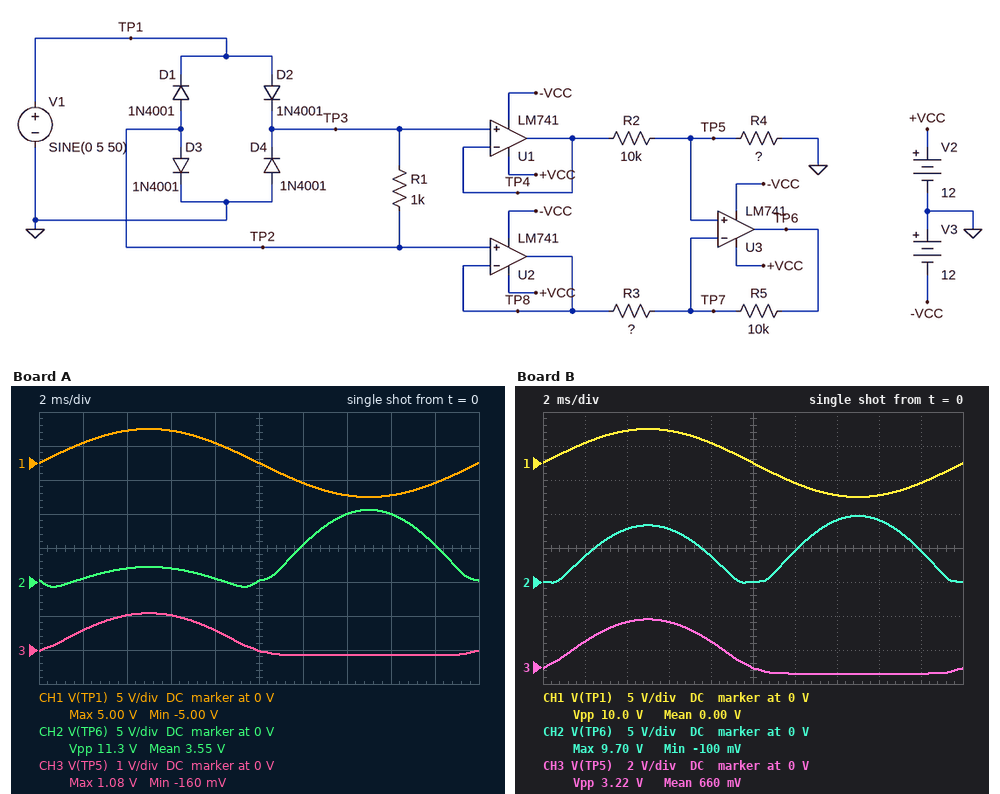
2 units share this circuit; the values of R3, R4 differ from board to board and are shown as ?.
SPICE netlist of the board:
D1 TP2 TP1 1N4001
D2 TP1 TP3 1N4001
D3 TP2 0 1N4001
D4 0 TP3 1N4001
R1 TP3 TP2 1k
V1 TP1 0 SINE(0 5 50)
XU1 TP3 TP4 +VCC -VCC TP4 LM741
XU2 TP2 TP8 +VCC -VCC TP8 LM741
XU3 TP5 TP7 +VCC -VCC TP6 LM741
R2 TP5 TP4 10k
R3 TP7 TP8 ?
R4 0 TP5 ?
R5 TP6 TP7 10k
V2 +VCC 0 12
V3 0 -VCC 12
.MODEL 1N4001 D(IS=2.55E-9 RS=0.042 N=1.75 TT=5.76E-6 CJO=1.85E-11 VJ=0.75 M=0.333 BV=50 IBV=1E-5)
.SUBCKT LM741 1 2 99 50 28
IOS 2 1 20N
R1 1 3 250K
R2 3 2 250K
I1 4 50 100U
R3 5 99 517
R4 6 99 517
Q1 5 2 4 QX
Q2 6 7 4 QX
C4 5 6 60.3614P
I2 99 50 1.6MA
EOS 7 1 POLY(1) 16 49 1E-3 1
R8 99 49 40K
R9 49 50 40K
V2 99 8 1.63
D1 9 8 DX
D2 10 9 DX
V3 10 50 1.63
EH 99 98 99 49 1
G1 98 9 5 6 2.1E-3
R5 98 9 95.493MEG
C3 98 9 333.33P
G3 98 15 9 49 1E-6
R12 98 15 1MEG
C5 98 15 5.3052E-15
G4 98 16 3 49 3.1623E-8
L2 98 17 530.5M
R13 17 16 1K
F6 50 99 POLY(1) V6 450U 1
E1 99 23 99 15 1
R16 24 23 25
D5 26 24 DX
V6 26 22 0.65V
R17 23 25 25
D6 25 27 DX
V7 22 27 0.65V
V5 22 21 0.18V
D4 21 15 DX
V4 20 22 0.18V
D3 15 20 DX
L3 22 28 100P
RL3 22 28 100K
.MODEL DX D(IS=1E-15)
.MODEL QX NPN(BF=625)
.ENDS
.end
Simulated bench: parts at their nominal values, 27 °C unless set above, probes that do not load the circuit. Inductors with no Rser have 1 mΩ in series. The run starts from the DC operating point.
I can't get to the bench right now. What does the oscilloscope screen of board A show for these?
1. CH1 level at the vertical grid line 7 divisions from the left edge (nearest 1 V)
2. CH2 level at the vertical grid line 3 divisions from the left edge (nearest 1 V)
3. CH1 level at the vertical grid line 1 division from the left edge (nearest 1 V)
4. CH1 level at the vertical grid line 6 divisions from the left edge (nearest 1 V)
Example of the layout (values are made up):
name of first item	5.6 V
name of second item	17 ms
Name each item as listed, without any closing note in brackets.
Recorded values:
CH1 level at the vertical grid line 7 divisions from the left edge	-5 V
CH2 level at the vertical grid line 3 divisions from the left edge	2 V
CH1 level at the vertical grid line 1 division from the left edge	3 V
CH1 level at the vertical grid line 6 divisions from the left edge	-3 V
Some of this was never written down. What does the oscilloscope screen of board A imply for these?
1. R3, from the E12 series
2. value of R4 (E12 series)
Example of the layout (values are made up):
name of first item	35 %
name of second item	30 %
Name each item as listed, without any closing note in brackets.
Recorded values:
R3, from the E12 series	3.9 kΩ
value of R4	3.3 kΩ
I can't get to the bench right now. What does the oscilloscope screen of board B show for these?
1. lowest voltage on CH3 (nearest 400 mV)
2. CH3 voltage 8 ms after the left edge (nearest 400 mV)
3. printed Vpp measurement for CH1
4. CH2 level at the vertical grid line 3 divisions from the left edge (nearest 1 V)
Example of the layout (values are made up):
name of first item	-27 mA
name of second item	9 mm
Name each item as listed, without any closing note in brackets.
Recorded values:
lowest voltage on CH3	-400 mV
CH3 voltage 8 ms after the left edge	1.6 V
printed Vpp measurement for CH1	10.0 V
CH2 level at the vertical grid line 3 divisions from the left edge	8 V
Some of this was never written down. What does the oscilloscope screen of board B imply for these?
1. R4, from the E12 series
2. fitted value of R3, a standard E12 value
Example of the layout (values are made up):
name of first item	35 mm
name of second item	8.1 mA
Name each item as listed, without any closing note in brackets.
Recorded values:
R4, from the E12 series	18 kΩ
fitted value of R3, a standard E12 value	3.9 kΩ
